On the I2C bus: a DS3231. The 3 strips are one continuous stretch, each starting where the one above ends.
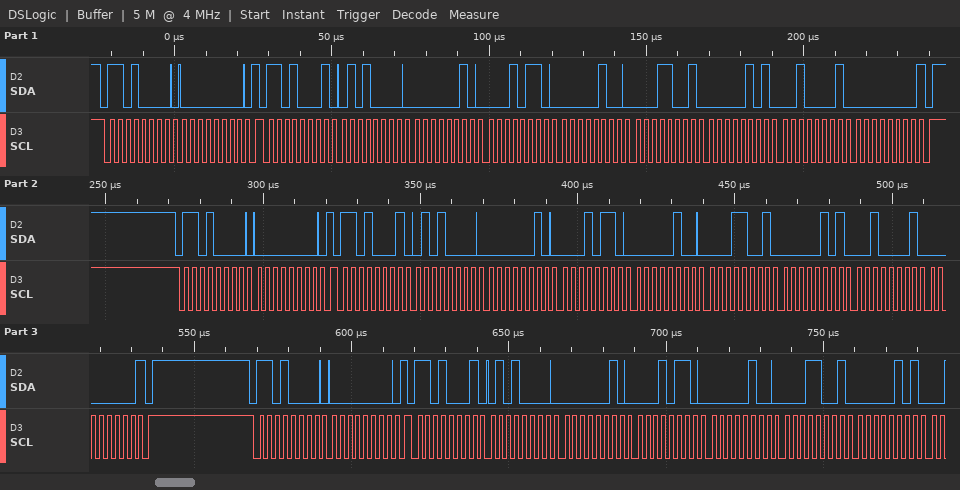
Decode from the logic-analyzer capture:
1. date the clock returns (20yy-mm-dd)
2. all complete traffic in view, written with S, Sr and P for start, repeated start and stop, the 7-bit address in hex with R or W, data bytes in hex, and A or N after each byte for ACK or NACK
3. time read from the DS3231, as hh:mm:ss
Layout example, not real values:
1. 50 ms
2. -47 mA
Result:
1. 2021-05-19
2. S 68W A 00 A Sr 68R A 50 A 02 A 16 A 04 A 19 A 05 A 21 A 00 N P S 68W A 00 A Sr 68R A 50 A 02 A 16 A 04 A 19 A 05 A 21 A 00 N P S 68W A 00 A Sr 68R A 50 A 02 A 16 A 04 A 19 A 05 A
3. 16:02:50
